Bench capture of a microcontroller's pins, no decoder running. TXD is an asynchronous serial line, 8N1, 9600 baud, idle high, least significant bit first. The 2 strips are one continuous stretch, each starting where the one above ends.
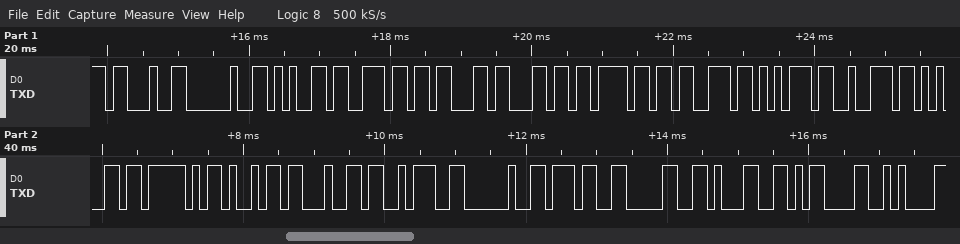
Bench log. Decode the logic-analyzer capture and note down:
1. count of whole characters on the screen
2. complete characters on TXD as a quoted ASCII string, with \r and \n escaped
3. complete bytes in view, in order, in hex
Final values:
21
"# enclosure_id: 701\r\n"
0x23 0x20 0x65 0x6E 0x63 0x6C 0x6F 0x73 0x75 0x72 0x65 0x5F 0x69 0x64 0x3A 0x20 0x37 0x30 0x31 0x0D 0x0A
